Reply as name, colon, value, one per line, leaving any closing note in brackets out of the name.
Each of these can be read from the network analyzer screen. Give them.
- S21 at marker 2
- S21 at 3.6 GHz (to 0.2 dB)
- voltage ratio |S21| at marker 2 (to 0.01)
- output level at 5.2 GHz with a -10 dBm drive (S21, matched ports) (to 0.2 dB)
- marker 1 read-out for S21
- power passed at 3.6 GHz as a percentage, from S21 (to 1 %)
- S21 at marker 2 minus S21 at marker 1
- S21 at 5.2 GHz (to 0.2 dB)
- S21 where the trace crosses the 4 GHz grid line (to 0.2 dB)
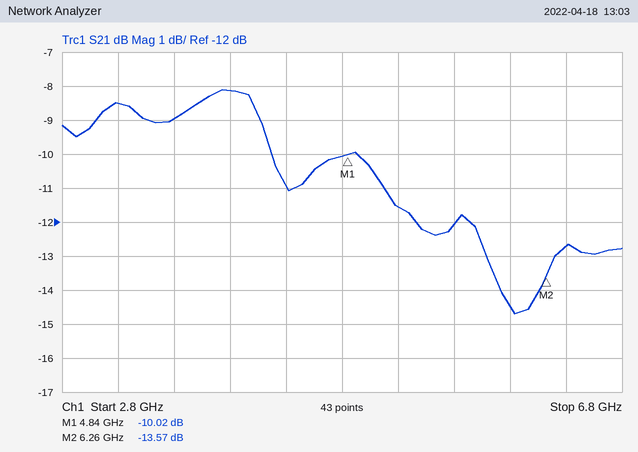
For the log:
S21 at marker 2: -13.57 dB
S21 at 3.6 GHz: -9.0 dB
voltage ratio |S21| at marker 2: 0.21
output level at 5.2 GHz with a -10 dBm drive (S21, matched ports): -21.6 dBm
marker 1 read-out for S21: -10.02 dB
power passed at 3.6 GHz as a percentage, from S21: 13 %
S21 at marker 2 minus S21 at marker 1: -3.55 dB
S21 at 5.2 GHz: -11.6 dB
S21 where the trace crosses the 4 GHz grid line: -8.2 dB
